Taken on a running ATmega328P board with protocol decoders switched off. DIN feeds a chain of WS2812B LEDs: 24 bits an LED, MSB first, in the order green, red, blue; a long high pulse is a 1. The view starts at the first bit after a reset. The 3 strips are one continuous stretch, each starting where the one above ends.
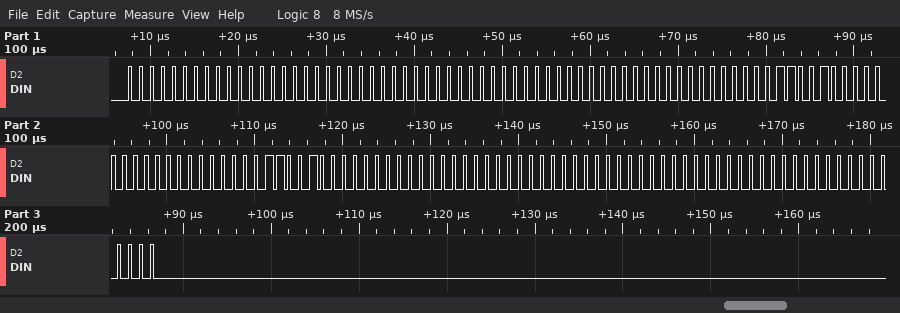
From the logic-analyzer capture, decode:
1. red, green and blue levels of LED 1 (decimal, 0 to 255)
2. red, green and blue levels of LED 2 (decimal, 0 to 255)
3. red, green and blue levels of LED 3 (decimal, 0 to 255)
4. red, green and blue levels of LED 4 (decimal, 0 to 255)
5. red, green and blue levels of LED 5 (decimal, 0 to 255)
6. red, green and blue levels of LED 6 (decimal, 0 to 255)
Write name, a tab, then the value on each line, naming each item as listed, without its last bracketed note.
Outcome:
red, green and blue levels of LED 1	0, 0, 0
red, green and blue levels of LED 2	0, 0, 0
red, green and blue levels of LED 3	25, 0, 0
red, green and blue levels of LED 4	25, 0, 0
red, green and blue levels of LED 5	0, 0, 0
red, green and blue levels of LED 6	0, 0, 0
